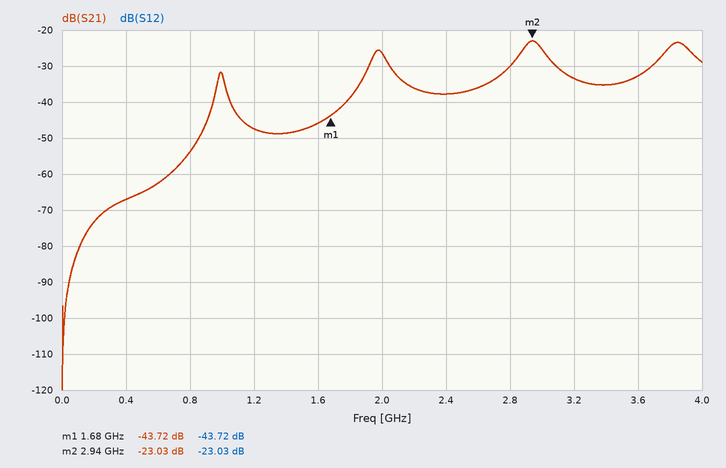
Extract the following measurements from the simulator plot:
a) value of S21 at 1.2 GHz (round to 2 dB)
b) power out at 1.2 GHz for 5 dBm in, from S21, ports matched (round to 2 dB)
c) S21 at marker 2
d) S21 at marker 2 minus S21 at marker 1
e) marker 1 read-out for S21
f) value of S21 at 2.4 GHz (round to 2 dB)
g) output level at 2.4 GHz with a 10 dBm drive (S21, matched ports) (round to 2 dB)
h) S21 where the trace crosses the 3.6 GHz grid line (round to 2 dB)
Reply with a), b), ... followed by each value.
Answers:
a) -48 dB
b) -42 dBm
c) -23.03 dB
d) 20.69 dB
e) -43.72 dB
f) -38 dB
g) -28 dBm
h) -32 dB
